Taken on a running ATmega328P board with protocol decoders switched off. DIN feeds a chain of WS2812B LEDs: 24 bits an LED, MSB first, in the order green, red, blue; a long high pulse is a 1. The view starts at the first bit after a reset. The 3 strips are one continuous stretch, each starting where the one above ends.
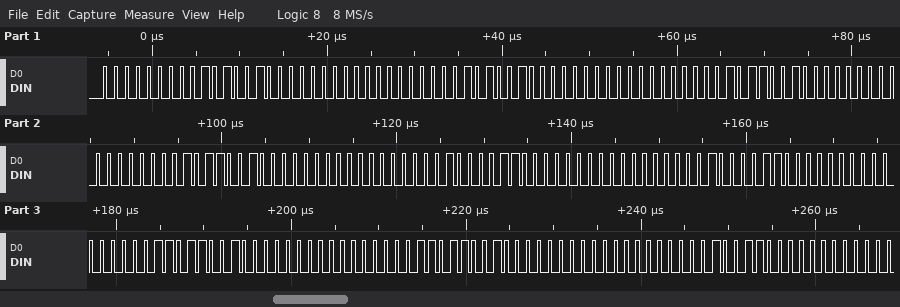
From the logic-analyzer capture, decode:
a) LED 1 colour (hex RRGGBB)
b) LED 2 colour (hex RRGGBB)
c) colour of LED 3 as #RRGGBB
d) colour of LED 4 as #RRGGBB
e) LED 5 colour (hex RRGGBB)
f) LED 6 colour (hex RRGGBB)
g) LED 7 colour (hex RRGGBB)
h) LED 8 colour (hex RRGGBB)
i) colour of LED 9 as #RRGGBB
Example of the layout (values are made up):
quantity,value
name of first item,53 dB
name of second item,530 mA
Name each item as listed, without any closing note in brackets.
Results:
quantity,value
LED 1 colour,#520000
LED 2 colour,#520000
colour of LED 3 as #RRGGBB,#590000
colour of LED 4 as #RRGGBB,#590000
LED 5 colour,#430000
LED 6 colour,#430000
LED 7 colour,#D90000
LED 8 colour,#D90000
colour of LED 9 as #RRGGBB,#130000
